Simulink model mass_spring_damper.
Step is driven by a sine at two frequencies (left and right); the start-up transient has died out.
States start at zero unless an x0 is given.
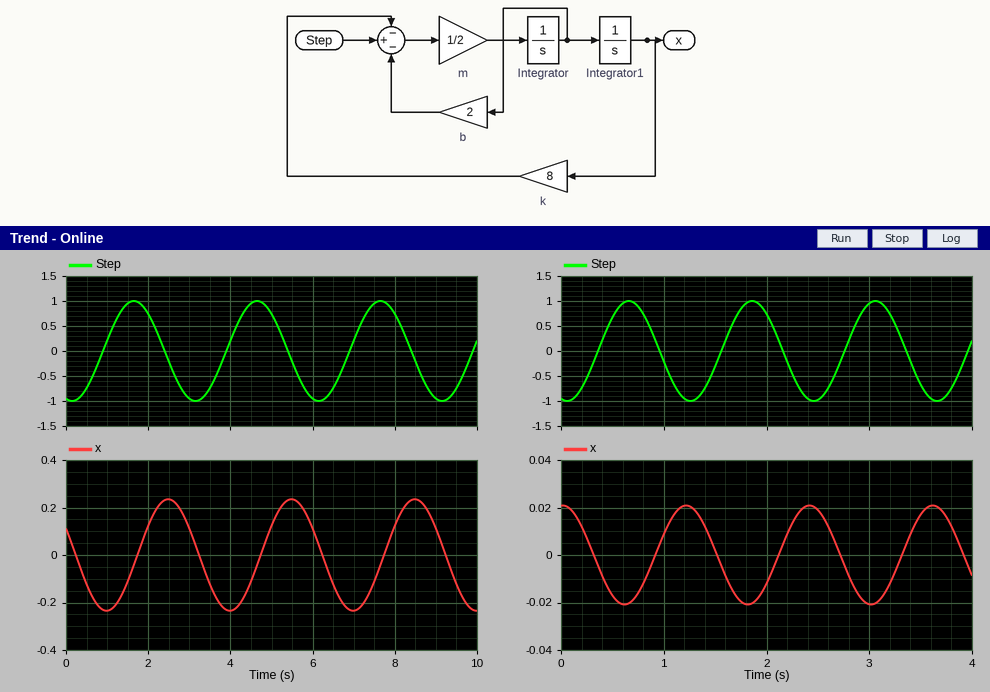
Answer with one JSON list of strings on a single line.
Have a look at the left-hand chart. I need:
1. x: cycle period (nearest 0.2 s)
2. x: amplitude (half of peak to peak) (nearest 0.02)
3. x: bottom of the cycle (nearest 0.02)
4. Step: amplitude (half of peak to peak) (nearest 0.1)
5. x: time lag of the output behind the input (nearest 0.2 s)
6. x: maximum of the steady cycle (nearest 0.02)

["3.0 s", "0.24", "-0.24", "1.0", "0.8 s", "0.24"]
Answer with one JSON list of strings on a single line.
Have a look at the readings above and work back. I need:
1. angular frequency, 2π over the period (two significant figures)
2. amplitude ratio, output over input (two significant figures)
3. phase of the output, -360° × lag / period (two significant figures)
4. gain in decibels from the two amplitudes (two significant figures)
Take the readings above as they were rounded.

["2.1 rad/s", "0.24", "-96°", "-12 dB"]
